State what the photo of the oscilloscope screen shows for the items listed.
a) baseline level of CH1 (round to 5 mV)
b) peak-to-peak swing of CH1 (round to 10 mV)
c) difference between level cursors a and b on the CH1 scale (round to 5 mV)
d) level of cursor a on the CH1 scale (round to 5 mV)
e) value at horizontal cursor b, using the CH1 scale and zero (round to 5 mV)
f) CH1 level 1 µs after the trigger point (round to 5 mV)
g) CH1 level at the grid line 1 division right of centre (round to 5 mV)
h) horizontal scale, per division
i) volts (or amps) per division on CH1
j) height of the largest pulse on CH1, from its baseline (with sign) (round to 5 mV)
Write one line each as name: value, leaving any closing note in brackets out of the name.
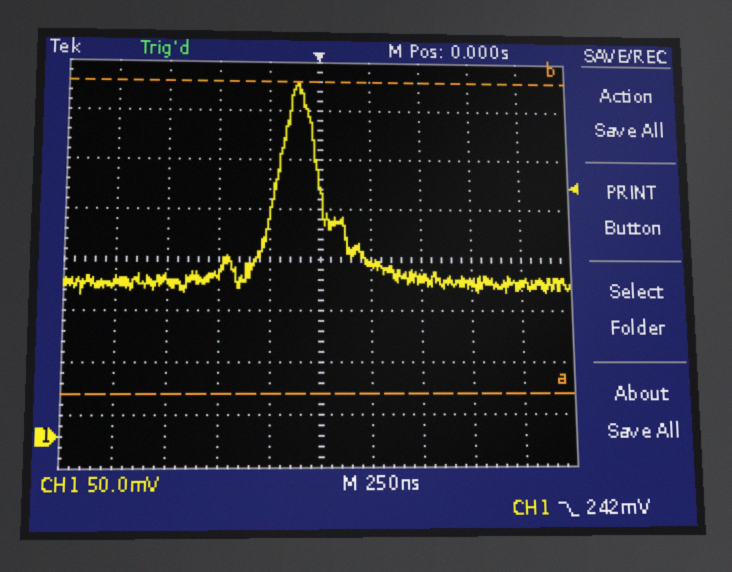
baseline level of CH1: 150 mV
peak-to-peak swing of CH1: 210 mV
difference between level cursors a and b on the CH1 scale: 310 mV
level of cursor a on the CH1 scale: 40 mV
value at horizontal cursor b, using the CH1 scale and zero: 350 mV
CH1 level 1 µs after the trigger point: 145 mV
CH1 level at the grid line 1 division right of centre: 165 mV
horizontal scale, per division: 250 ns
volts (or amps) per division on CH1: 50 mV
height of the largest pulse on CH1, from its baseline (with sign): +200 mV
